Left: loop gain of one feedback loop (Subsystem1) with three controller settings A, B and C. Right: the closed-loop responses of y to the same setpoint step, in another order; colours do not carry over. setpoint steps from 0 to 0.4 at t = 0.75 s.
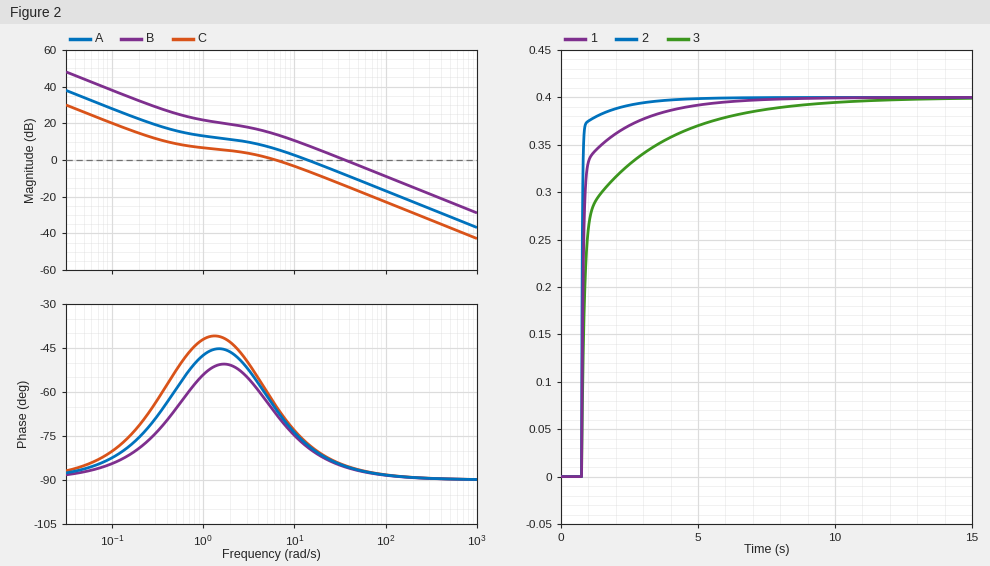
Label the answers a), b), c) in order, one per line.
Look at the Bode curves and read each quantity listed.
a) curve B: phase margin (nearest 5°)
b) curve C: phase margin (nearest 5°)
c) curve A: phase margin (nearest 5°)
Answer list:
a) 95°
b) 115°
c) 100°
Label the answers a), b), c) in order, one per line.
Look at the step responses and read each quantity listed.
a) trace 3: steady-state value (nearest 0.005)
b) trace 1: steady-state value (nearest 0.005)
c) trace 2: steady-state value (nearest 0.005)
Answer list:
a) 0.400
b) 0.400
c) 0.400
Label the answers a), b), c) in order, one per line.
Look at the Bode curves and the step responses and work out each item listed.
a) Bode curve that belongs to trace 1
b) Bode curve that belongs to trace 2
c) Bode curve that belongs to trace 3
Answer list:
a) A
b) B
c) C
